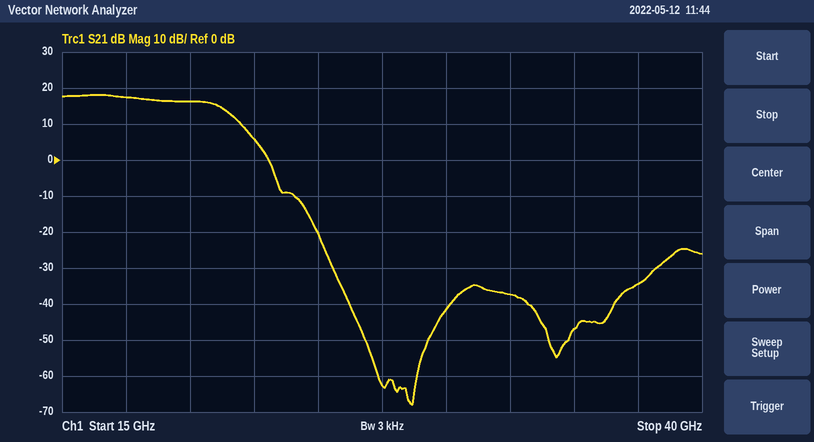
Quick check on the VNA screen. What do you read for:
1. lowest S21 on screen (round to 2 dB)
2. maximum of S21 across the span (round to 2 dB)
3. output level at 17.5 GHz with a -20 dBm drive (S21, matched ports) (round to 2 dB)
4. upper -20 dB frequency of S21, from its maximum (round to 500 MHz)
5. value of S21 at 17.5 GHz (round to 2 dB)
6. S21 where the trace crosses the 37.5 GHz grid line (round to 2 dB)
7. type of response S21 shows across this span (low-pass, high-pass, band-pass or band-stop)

-68 dB
18 dB
-2 dBm
23.0 GHz
18 dB
-34 dB
low-pass
